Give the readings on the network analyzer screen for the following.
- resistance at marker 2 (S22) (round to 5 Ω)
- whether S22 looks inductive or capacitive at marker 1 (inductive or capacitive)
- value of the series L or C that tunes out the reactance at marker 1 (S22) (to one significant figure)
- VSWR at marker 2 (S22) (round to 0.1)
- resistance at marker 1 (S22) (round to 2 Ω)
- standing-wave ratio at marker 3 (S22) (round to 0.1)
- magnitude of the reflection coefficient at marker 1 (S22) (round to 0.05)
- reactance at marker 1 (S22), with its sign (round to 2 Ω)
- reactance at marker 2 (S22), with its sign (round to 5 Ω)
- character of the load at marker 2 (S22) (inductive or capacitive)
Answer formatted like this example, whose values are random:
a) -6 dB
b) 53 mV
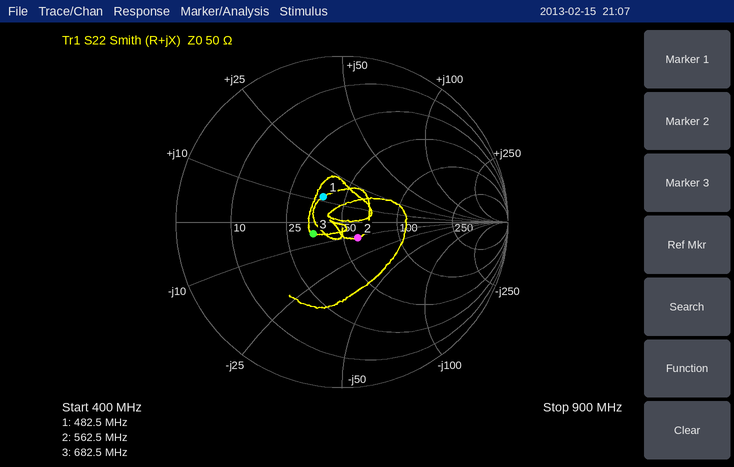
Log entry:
a) 60 Ω
b) inductive
c) 30 pF
d) 1.3
e) 38 Ω
f) 1.5
g) 0.20
h) +12 Ω
i) -10 Ω
j) capacitive
